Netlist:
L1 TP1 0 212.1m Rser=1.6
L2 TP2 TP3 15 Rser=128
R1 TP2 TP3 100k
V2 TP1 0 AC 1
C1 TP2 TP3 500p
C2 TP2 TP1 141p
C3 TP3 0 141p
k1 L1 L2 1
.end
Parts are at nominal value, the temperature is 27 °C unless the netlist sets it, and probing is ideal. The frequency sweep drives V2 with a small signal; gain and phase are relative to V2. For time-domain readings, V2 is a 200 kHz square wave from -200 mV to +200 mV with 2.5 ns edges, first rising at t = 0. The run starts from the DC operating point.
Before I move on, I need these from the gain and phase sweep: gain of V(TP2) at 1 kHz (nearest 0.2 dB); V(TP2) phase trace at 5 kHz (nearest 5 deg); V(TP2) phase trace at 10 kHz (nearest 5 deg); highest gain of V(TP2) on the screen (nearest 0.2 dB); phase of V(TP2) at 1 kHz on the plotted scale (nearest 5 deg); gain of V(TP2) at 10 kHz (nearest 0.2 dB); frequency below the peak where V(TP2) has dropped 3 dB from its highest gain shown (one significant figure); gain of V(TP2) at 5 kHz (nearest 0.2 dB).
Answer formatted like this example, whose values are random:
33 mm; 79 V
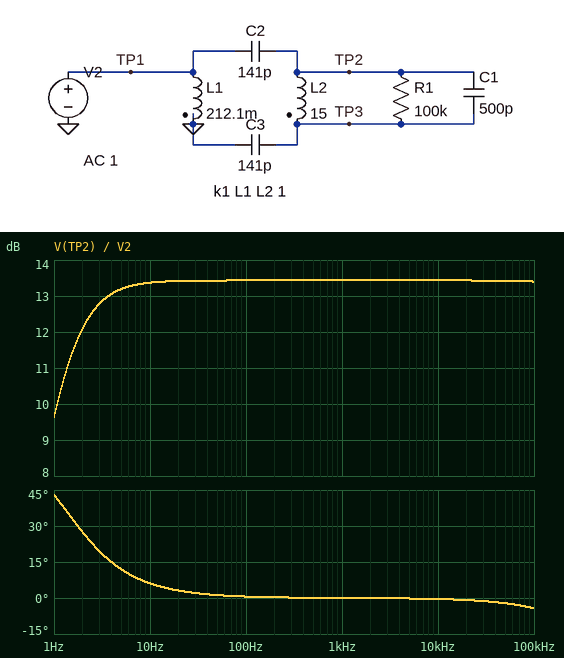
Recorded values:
13.4 dB; 0 deg; 0 deg; 13.4 dB; 0 deg; 13.4 dB; 1 Hz; 13.4 dB
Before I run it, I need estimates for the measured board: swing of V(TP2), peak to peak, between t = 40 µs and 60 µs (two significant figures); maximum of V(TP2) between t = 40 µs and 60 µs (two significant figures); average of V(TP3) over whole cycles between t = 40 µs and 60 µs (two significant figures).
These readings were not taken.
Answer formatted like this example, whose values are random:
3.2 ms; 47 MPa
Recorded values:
1.9 V; 1.9 V; -740 mV
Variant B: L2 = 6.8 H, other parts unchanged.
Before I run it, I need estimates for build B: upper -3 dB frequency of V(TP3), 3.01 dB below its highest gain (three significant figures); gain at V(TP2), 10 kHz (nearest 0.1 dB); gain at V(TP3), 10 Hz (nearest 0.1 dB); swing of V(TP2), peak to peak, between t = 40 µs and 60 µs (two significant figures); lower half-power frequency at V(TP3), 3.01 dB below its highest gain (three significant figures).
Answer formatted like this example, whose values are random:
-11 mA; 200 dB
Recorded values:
1.62 MHz; 10.4 dB; 7.3 dB; 1.3 V; 1.14 Hz
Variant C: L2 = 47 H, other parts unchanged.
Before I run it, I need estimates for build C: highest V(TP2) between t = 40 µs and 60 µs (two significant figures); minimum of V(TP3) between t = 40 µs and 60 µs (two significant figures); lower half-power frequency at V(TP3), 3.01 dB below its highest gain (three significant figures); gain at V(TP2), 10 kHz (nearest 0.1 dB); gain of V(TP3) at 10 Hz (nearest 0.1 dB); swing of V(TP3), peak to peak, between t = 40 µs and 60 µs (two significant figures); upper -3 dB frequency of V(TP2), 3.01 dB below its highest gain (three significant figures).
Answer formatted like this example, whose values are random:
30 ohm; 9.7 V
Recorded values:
3.2 V; -2.9 V; 1.19 Hz; 18.0 dB; 16.7 dB; 3.1 V; 584 kHz
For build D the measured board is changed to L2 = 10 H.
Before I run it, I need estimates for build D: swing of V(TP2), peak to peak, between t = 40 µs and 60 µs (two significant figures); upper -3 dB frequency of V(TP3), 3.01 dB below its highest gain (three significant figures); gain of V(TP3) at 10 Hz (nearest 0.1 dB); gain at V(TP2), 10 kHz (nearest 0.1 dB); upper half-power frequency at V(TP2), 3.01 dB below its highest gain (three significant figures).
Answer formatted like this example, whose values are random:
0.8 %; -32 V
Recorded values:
1.6 V; 1.41 MHz; 9.3 dB; 11.9 dB; 1.40 MHz
